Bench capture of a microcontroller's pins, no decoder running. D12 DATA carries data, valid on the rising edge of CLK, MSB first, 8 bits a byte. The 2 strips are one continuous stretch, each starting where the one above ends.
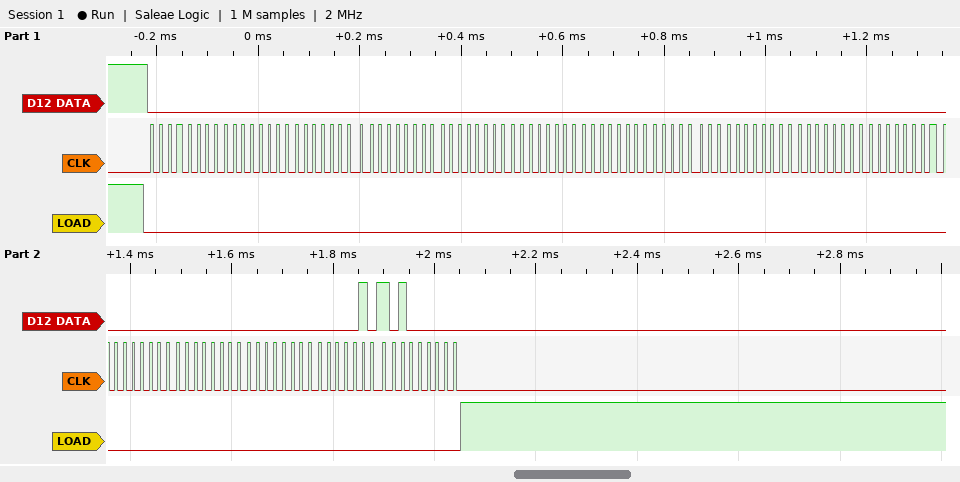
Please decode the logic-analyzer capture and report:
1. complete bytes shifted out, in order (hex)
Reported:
00 00 00 00 00 00 00 00 00 00 00 00 00 00 05 40
